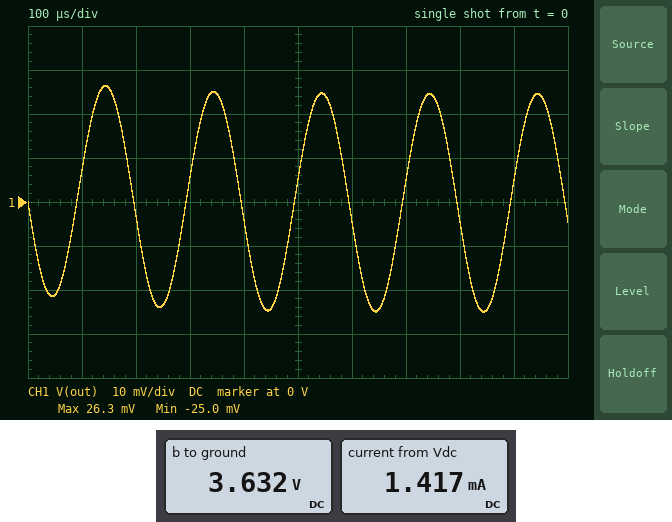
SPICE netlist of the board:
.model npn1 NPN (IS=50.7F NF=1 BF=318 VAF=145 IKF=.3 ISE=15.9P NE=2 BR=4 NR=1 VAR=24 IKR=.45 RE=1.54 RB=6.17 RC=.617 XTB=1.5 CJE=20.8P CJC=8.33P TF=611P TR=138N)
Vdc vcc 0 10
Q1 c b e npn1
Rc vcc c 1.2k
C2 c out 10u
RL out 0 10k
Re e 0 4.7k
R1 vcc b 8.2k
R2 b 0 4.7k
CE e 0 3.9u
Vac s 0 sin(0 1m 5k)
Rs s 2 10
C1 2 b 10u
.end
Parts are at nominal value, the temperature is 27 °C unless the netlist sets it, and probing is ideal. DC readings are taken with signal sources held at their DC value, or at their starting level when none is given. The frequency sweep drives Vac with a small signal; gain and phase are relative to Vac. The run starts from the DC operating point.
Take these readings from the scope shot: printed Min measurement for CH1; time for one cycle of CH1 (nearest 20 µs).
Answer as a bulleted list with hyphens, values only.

- -25.0 mV
- 200 µs
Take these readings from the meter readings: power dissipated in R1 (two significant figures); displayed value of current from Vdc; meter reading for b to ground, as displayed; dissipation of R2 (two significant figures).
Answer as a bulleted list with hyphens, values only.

- 4.9 mW
- 1.417 mA
- 3.632 V
- 2.8 mW
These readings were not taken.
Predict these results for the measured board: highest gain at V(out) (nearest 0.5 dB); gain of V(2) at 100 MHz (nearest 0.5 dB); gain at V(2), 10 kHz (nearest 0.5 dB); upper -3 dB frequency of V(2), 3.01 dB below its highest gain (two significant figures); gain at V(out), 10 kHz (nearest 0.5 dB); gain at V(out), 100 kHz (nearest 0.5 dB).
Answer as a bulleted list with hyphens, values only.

- 28.0 dB
- -2.0 dB
- 0 dB
- 200 MHz
- 28.0 dB
- 28.0 dB
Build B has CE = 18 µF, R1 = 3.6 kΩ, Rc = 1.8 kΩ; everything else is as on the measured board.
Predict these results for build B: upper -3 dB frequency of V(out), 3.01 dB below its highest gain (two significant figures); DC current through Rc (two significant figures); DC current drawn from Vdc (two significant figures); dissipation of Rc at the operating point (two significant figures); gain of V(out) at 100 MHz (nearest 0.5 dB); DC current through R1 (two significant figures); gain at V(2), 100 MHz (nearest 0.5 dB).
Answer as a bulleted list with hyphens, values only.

- 12 MHz
- 1.1 mA
- 2.3 mA
- 2.0 mW
- 16.5 dB
- 1.2 mA
- -3.0 dB
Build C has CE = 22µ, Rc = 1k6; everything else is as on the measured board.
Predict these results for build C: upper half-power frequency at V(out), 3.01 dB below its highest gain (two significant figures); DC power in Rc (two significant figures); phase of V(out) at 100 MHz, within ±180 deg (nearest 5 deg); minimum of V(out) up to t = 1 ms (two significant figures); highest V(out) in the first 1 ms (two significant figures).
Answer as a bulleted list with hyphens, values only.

- 19 MHz
- 660 µW
- 75 deg
- -32 mV
- 33 mV
